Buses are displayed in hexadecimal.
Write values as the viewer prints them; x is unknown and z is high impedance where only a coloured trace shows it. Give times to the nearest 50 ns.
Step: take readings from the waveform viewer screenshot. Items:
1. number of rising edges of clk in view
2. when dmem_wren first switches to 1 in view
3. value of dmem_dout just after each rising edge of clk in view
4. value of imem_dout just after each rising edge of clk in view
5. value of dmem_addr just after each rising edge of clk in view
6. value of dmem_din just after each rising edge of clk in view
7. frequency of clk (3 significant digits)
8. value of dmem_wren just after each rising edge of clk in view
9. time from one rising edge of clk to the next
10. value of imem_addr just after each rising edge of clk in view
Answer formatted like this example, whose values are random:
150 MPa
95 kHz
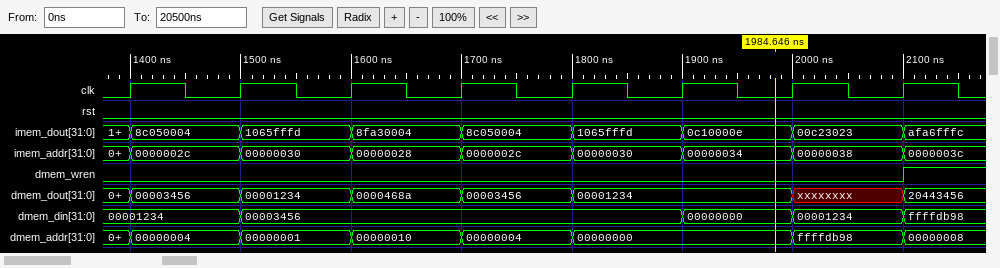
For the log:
8
2100 ns
00003456, 00001234, 0000468a, 00003456, 00001234, 00001234, xxxxxxxx, 20443456
8c050004, 1065fffd, 8fa30004, 8c050004, 1065fffd, 0c10000e, 00c23023, afa6fffc
00000004, 00000001, 00000010, 00000004, 00000000, 00000000, ffffdb98, 00000008
00001234, 00003456, 00003456, 00003456, 00003456, 00000000, 00001234, ffffdb98
10.0 MHz
0 0 0 0 0 0 0 1
100 ns
0000002c, 00000030, 00000028, 0000002c, 00000030, 00000034, 00000038, 0000003c
